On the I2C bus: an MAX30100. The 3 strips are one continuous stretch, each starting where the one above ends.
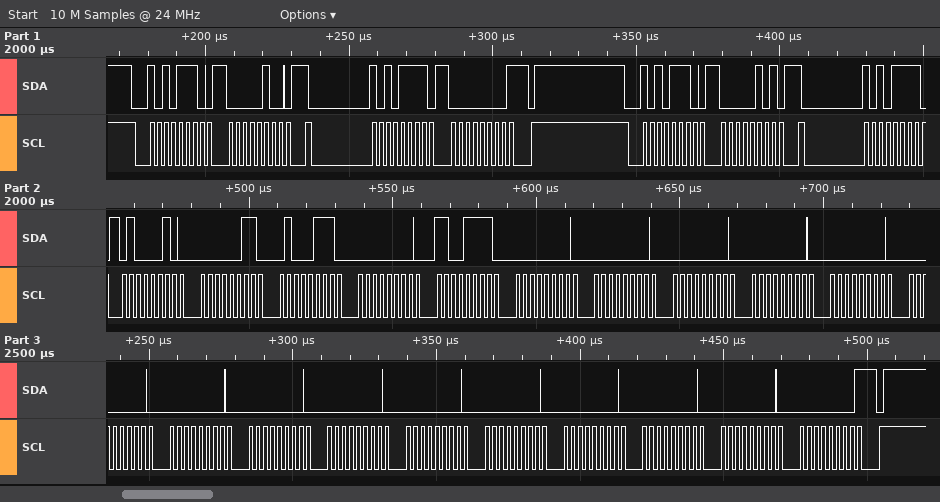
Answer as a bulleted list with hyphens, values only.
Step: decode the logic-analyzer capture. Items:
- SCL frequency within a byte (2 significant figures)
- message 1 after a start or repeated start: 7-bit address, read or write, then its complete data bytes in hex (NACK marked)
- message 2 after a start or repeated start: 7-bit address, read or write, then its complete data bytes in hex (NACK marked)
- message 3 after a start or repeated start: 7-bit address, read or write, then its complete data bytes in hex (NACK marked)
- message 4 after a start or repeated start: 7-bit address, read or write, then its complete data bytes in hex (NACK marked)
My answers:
- 400 kHz
- 0x57 write: 04
- 0x57 read: 00 NACK
- 0x57 write: 05
- 0x57 read: 42 03 47 00 CF 00 00 00 00 00 00 00 00 00 00 00 00 00 00 00 NACK
